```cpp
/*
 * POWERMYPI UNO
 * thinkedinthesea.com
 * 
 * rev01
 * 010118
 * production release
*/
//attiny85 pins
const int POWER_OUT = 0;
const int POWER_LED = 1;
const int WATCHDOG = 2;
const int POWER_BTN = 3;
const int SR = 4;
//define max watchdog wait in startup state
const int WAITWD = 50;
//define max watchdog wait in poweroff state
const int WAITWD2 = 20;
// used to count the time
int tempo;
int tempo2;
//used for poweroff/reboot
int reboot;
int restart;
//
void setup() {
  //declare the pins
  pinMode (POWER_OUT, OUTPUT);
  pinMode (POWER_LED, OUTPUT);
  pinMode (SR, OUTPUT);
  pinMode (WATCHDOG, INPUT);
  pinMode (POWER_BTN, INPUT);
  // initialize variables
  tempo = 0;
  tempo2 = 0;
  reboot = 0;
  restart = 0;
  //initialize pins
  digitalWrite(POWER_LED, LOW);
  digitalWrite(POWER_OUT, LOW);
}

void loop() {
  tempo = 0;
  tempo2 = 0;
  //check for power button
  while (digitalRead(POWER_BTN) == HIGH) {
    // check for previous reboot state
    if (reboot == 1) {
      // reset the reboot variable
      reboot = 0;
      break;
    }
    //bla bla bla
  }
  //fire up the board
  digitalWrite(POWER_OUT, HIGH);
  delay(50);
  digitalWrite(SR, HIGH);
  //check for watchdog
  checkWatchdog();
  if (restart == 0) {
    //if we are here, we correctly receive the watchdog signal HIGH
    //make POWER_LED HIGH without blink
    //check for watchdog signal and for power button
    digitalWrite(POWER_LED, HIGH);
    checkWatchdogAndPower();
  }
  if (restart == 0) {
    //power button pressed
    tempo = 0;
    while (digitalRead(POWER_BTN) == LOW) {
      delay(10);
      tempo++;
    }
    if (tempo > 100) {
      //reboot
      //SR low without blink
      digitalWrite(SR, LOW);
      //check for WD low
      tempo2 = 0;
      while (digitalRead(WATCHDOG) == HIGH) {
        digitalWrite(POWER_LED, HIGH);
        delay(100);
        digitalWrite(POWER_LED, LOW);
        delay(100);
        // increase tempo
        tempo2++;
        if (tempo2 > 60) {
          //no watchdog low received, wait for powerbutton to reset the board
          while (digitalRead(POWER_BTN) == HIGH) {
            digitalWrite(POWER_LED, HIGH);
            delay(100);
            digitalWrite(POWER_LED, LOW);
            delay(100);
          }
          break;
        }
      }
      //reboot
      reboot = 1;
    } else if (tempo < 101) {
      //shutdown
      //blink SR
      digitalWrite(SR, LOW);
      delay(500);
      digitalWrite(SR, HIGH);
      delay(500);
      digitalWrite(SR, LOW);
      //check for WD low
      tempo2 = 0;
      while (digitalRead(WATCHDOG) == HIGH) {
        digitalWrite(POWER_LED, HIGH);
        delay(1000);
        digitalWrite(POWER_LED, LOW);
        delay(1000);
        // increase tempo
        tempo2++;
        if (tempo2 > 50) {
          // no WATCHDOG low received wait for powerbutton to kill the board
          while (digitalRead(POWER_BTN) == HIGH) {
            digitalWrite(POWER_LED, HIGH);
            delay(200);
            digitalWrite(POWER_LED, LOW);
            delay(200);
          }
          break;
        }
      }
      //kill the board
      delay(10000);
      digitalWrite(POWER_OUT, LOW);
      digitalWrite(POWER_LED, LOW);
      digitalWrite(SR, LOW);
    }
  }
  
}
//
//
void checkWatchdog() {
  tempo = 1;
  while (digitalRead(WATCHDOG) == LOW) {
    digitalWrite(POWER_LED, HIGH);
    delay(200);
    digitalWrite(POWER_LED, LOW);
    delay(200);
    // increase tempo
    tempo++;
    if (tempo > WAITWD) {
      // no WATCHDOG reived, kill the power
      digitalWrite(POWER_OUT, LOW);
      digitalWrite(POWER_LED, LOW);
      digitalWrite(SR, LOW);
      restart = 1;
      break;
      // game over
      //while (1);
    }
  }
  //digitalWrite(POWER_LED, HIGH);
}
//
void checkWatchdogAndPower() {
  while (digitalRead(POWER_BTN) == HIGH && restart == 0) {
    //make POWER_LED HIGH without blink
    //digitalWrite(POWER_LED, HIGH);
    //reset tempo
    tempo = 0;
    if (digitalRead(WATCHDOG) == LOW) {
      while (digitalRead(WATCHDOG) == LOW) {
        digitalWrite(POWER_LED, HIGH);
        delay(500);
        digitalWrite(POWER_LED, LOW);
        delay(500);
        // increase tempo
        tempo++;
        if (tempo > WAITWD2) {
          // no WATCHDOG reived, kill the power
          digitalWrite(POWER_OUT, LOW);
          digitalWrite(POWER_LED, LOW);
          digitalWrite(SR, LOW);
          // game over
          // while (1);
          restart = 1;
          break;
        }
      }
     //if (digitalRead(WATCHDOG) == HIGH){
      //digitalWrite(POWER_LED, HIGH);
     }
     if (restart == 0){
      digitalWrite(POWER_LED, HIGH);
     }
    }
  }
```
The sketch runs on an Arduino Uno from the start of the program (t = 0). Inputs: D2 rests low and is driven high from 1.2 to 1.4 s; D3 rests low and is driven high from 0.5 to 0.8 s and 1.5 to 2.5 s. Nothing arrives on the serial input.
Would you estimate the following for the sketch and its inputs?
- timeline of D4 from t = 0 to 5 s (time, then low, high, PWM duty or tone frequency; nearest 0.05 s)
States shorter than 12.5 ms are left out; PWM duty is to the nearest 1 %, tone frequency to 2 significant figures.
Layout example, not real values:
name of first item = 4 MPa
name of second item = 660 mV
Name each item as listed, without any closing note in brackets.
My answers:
timeline of D4 from t = 0 to 5 s = 0 s low; 0.05 s high; 1.5 s low; 2 s high; 2.5 s low
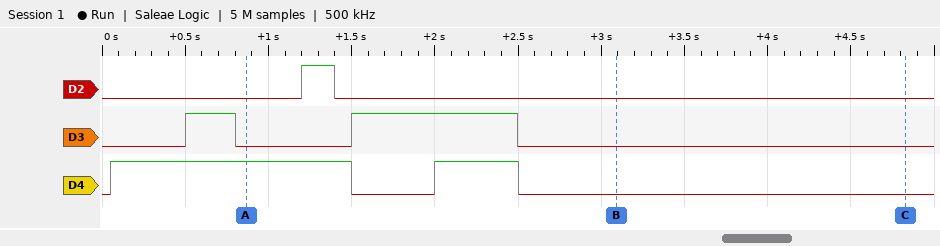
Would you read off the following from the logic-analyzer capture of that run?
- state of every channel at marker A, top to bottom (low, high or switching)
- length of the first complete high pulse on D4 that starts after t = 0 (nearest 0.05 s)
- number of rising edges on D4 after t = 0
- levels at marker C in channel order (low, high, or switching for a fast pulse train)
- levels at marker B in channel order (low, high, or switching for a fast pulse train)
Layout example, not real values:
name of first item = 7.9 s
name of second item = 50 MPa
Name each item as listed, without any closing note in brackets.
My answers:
state of every channel at marker A, top to bottom = D2 low, D3 low, D4 high
length of the first complete high pulse on D4 that starts after t = 0 = 1.45 s
number of rising edges on D4 after t = 0 = 2
levels at marker C in channel order = D2 low, D3 low, D4 low
levels at marker B in channel order = D2 low, D3 low, D4 low
